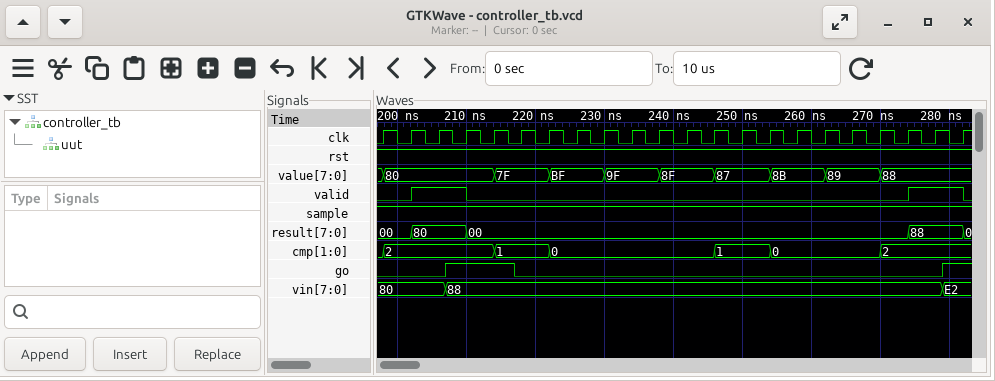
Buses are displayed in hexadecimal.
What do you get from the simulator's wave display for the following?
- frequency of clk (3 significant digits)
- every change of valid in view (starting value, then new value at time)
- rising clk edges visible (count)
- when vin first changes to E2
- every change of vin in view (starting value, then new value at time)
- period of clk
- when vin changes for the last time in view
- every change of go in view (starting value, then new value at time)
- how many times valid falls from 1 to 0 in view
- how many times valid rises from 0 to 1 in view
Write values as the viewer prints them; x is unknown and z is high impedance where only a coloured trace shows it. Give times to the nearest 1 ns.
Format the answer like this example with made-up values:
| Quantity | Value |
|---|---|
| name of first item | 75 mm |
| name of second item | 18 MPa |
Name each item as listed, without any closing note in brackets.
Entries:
| Quantity | Value |
|---|---|
| frequency of clk | 250 MHz |
| every change of valid in view | 0, 1 at 202 ns, 0 at 210 ns, 1 at 274 ns, 0 at 282 ns |
| rising clk edges visible | 22 |
| when vin first changes to E2 | 279 ns |
| every change of vin in view | 80, 88 at 207 ns, E2 at 279 ns |
| period of clk | 4 ns |
| when vin changes for the last time in view | 279 ns |
| every change of go in view | 0, 1 at 207 ns, 0 at 217 ns, 1 at 279 ns |
| how many times valid falls from 1 to 0 in view | 2 |
| how many times valid rises from 0 to 1 in view | 2 |
